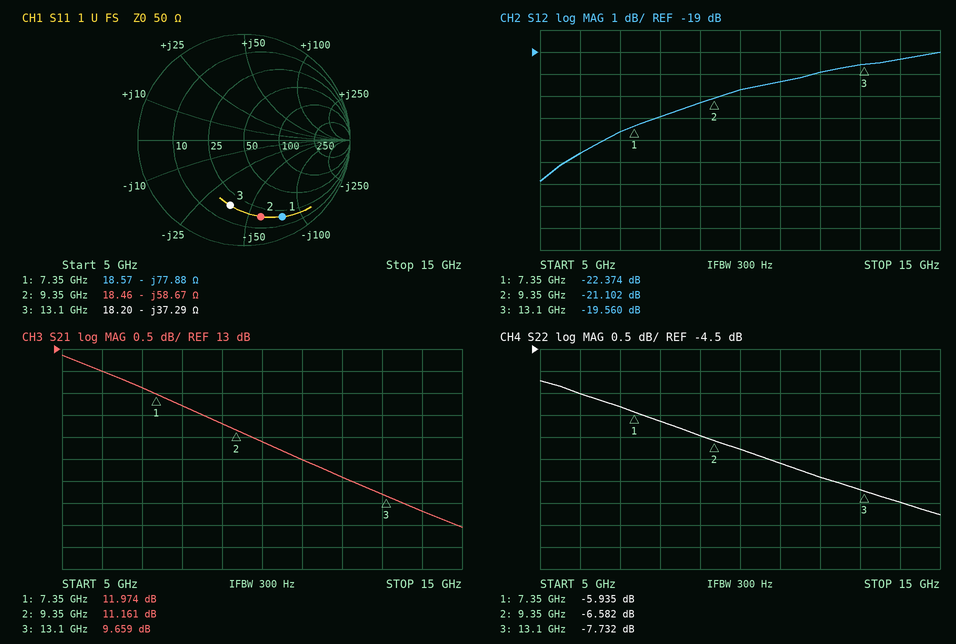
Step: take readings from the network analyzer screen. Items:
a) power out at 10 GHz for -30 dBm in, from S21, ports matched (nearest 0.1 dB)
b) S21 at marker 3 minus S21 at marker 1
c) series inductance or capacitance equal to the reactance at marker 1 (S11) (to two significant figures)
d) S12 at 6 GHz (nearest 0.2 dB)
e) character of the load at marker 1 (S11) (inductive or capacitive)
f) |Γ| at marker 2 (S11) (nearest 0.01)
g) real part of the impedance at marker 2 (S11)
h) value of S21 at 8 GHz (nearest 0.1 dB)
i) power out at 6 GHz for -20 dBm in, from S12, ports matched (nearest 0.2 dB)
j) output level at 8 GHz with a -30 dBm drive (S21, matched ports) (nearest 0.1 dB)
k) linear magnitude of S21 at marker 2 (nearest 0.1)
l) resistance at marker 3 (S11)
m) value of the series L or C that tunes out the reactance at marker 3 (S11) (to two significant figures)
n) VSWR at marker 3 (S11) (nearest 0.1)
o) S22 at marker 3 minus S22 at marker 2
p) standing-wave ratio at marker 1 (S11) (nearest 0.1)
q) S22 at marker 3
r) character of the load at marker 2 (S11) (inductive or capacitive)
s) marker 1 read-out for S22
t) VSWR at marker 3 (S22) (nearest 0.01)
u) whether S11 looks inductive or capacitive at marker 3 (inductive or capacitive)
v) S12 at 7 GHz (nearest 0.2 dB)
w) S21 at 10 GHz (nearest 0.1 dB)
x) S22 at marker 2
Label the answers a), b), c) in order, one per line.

a) -19.1 dBm
b) -2.315 dB
c) 280 fF
d) -23.6 dB
e) capacitive
f) 0.74
g) 18.46 Ω
h) 11.7 dB
i) -43.6 dBm
j) -18.3 dBm
k) 3.6
l) 18.20 Ω
m) 450 pH
n) 4.4
o) -1.150 dB
p) 9.5
q) -7.732 dB
r) capacitive
s) -5.935 dB
t) 2.39
u) capacitive
v) -22.6 dB
w) 10.9 dB
x) -6.582 dB
